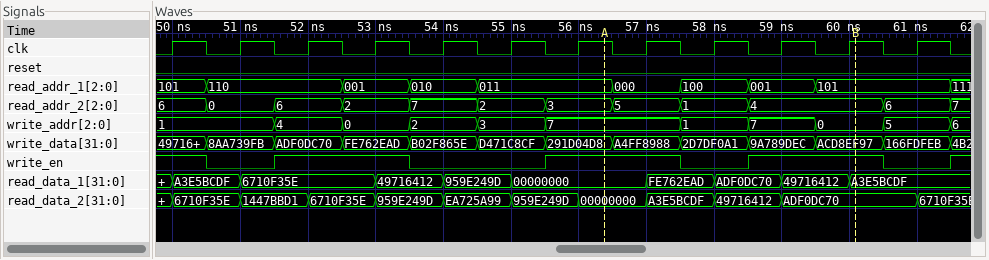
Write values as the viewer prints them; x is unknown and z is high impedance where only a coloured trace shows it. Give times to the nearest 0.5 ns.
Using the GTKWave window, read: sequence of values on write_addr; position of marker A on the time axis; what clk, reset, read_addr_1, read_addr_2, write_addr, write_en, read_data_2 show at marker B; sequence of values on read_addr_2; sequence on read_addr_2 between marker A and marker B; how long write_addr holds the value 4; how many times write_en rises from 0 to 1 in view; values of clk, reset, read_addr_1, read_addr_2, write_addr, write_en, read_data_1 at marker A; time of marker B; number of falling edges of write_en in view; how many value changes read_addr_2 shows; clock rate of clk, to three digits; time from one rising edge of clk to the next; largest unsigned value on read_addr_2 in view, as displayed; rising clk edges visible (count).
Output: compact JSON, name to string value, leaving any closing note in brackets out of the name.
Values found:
{"sequence of values on write_addr": "1, 4, 0, 2, 3, 7, 1, 7, 0, 5, 6", "position of marker A on the time axis": "56.5 ns", "what clk, reset, read_addr_1, read_addr_2, write_addr, write_en, read_data_2 show at marker B": "clk=1, reset=0, read_addr_1=101, read_addr_2=4, write_addr=0, write_en=1, read_data_2=ADF0DC70", "sequence of values on read_addr_2": "6, 0, 6, 2, 7, 2, 3, 5, 1, 4, 6, 7", "sequence on read_addr_2 between marker A and marker B": "3, 5, 1, 4", "how long write_addr holds the value 4": "1 ns", "how many times write_en rises from 0 to 1 in view": "4", "values of clk, reset, read_addr_1, read_addr_2, write_addr, write_en, read_data_1 at marker A": "clk=1, reset=0, read_addr_1=011, read_addr_2=3, write_addr=7, write_en=1, read_data_1=00000000", "time of marker B": "60 ns", "number of falling edges of write_en in view": "4", "how many value changes read_addr_2 shows": "11", "clock rate of clk, to three digits": "1.00 GHz", "time from one rising edge of clk to the next": "1 ns", "largest unsigned value on read_addr_2 in view, as displayed": "7", "rising clk edges visible": "12"}
